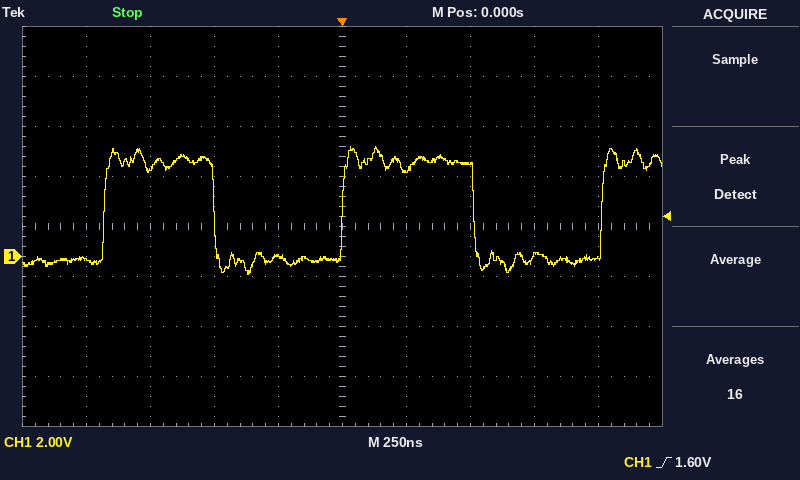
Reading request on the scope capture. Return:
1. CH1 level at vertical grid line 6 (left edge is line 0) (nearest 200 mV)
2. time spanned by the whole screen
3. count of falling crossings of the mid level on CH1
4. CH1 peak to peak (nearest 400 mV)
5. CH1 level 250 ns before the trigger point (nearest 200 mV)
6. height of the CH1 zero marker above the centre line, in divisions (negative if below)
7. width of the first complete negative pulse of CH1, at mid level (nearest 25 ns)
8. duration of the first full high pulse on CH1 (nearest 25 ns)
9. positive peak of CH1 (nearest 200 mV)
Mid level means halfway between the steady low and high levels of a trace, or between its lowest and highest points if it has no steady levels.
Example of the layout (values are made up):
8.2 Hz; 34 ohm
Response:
3.4 V; 2.5 µs; 2; 5.2 V; 0.0 V; -0.6 div; 500 ns; 425 ns; 4.4 V
